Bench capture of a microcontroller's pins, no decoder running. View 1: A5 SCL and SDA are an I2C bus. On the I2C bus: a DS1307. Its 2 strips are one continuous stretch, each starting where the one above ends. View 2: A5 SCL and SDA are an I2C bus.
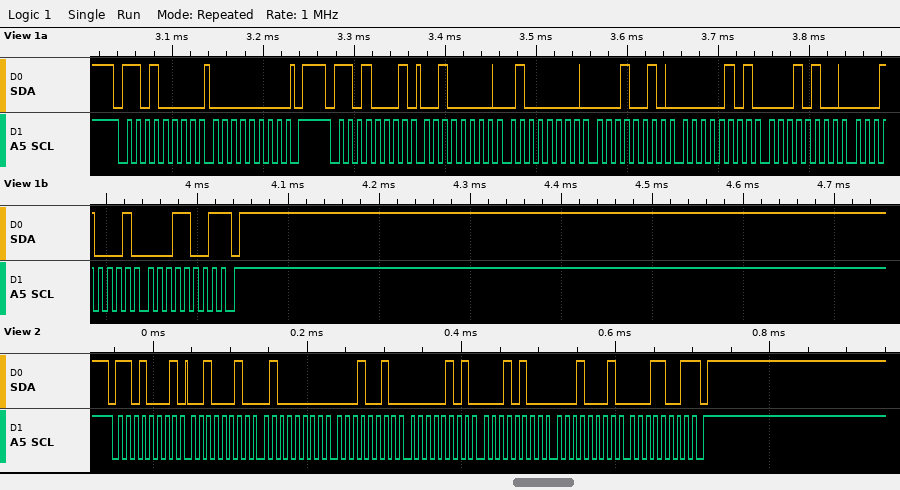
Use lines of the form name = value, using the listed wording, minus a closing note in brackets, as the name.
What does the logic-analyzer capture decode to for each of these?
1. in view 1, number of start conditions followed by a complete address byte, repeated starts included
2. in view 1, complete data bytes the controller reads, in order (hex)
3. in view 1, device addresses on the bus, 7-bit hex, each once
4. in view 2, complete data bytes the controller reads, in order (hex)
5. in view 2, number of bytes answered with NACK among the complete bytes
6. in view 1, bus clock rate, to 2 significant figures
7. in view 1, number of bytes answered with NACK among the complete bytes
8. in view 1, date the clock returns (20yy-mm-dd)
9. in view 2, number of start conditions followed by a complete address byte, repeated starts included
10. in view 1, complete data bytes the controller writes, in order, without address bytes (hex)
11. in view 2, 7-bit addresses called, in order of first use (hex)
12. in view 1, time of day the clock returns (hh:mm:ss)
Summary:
in view 1, number of start conditions followed by a complete address byte, repeated starts included = 2
in view 1, complete data bytes the controller reads, in order = 20 40 12 05 14 11 19
in view 1, device addresses on the bus, 7-bit hex, each once = 0x68
in view 2, complete data bytes the controller reads, in order = 22 40 12 05 14 11 19
in view 2, number of bytes answered with NACK among the complete bytes = 1
in view 1, bus clock rate, to 2 significant figures = 100 kHz
in view 1, number of bytes answered with NACK among the complete bytes = 1
in view 1, date the clock returns = 2019-11-14
in view 2, number of start conditions followed by a complete address byte, repeated starts included = 1
in view 1, complete data bytes the controller writes, in order, without address bytes = 00
in view 2, 7-bit addresses called, in order of first use = 0x68
in view 1, time of day the clock returns = 12:40:20
